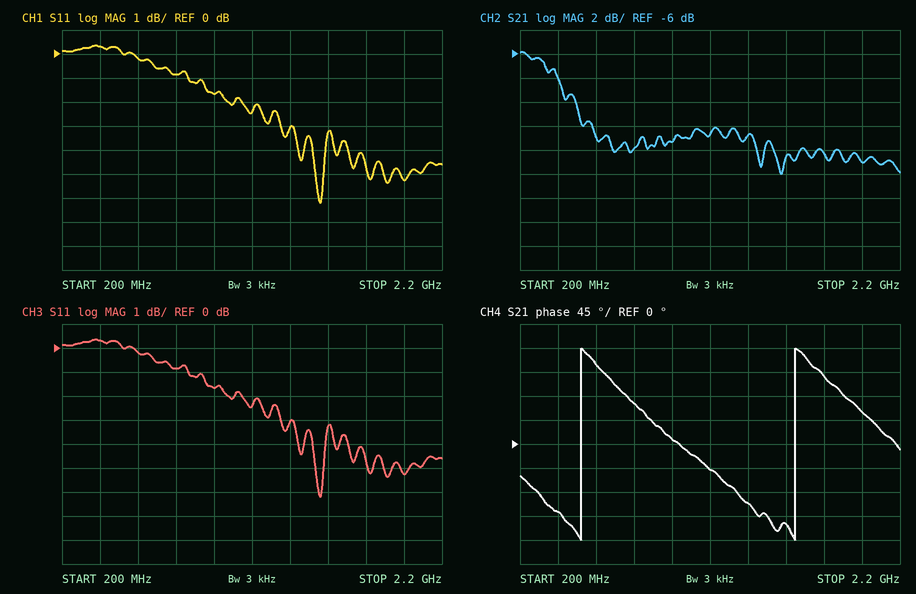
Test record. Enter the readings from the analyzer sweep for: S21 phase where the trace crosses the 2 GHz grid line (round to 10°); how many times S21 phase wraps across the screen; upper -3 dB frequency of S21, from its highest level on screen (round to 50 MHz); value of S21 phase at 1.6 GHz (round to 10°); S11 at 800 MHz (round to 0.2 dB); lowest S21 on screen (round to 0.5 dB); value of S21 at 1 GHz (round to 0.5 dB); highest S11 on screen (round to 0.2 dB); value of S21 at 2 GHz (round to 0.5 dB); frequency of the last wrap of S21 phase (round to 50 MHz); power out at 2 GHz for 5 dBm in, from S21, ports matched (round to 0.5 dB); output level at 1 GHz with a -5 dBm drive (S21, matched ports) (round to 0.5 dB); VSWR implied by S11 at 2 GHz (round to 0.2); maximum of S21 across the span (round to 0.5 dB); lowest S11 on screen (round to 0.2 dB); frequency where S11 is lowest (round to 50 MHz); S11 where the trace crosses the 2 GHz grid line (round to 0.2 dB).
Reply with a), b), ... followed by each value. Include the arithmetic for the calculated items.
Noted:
a) 60°
b) 2
c) 400 MHz
d) -150°
e) -0.8 dB
f) -16.0 dB
g) -13.5 dB
h) 0.4 dB
i) -15.0 dB
j) 1.65 GHz
k) 5 dBm + (-15.0 dB) = -10.0 dBm
l) -5 dBm + (-13.5 dB) = -18.5 dBm
m) |Γ| = 10^(-5.2/20) = 0.5495; VSWR = (1 + 0.5495)/(1 − 0.5495) ≈ 3.4
n) -6.0 dB
o) -6.2 dB
p) 1.55 GHz
q) -5.2 dB
